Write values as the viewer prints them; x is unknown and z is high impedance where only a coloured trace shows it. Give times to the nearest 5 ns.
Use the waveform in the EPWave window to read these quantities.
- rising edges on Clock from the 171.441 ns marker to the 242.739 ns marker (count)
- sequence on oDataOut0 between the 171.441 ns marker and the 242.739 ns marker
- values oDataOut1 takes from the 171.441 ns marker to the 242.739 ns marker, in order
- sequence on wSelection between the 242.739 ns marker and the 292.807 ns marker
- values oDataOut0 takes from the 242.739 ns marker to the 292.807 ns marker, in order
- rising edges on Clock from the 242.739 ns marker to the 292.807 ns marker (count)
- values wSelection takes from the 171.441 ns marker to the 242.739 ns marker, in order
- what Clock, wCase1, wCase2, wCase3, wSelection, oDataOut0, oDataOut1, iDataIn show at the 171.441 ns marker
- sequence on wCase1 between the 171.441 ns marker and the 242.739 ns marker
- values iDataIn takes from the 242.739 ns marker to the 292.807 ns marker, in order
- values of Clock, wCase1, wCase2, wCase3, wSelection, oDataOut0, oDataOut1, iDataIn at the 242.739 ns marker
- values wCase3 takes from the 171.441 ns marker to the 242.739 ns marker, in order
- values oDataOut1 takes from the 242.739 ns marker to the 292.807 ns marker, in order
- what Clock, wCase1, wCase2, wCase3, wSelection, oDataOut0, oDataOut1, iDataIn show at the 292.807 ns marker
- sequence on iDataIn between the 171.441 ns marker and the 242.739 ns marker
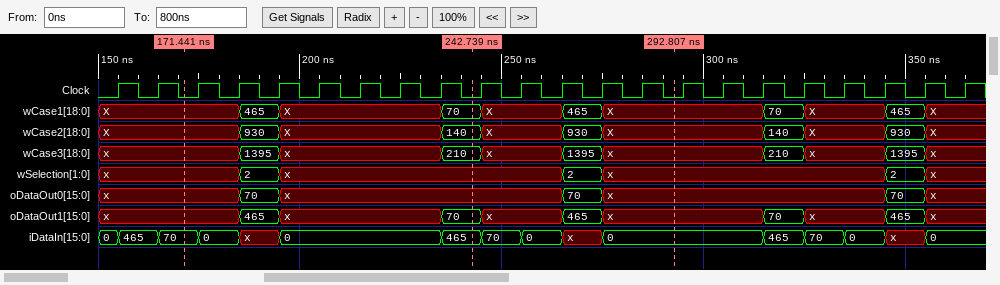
7
x, 70, x
x, 465, x, 70
x, 2, x
x, 70, x
5
x, 2, x
Clock=0, wCase1=X, wCase2=X, wCase3=x, wSelection=x, oDataOut0=x, oDataOut1=x, iDataIn=70
X, 465, X, 70
465, 70, 0, x, 0
Clock=0, wCase1=70, wCase2=140, wCase3=210, wSelection=x, oDataOut0=x, oDataOut1=70, iDataIn=465
x, 1395, x, 210
70, x, 465, x
Clock=0, wCase1=X, wCase2=X, wCase3=x, wSelection=x, oDataOut0=x, oDataOut1=x, iDataIn=0
70, 0, x, 0, 465
